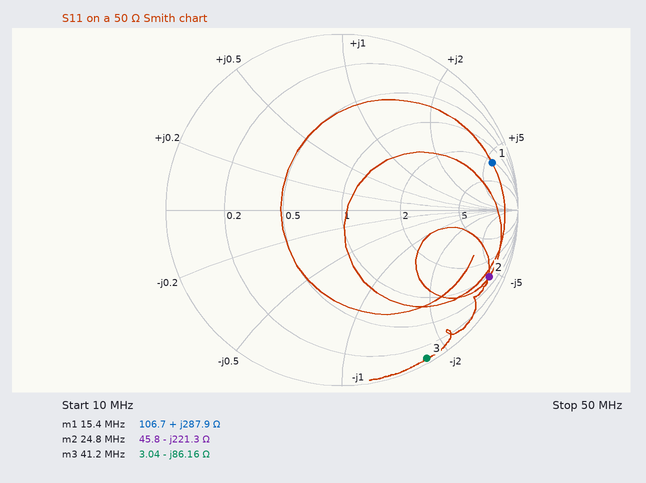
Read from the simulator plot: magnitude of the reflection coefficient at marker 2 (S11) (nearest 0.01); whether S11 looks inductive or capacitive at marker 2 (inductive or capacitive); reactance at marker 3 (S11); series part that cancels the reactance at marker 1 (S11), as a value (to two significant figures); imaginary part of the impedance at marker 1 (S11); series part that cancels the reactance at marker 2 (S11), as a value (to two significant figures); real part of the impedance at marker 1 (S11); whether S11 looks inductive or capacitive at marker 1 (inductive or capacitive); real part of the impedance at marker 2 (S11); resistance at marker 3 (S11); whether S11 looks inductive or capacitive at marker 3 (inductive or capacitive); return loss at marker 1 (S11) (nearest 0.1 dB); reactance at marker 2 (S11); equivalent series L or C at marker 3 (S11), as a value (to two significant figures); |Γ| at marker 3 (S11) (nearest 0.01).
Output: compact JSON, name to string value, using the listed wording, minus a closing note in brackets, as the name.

{"magnitude of the reflection coefficient at marker 2 (S11)": "0.92", "whether S11 looks inductive or capacitive at marker 2": "capacitive", "reactance at marker 3": "-86.16 Ω", "series part that cancels the reactance at marker 1 (S11), as a value": "36 pF", "imaginary part of the impedance at marker 1": "+287.9 Ω", "series part that cancels the reactance at marker 2 (S11), as a value": "1.4 µH", "real part of the impedance at marker 1": "106.7 Ω", "whether S11 looks inductive or capacitive at marker 1": "inductive", "real part of the impedance at marker 2": "45.8 Ω", "resistance at marker 3": "3.04 Ω", "whether S11 looks inductive or capacitive at marker 3": "capacitive", "return loss at marker 1 (S11)": "1.0 dB", "reactance at marker 2": "-221.3 Ω", "equivalent series L or C at marker 3 (S11), as a value": "45 pF", "|Γ| at marker 3 (S11)": "0.97"}
